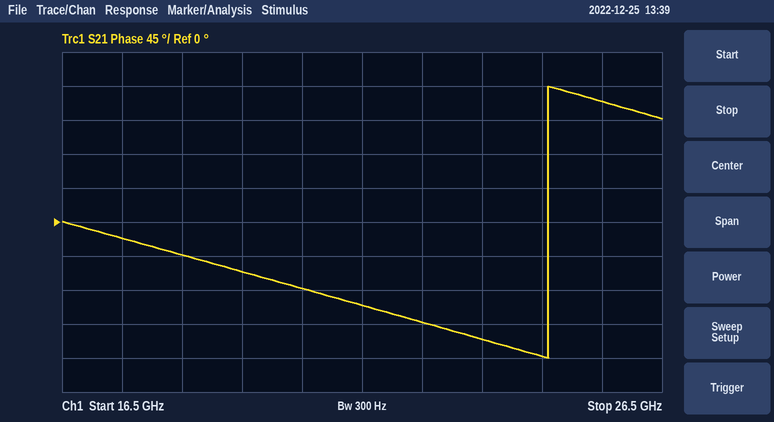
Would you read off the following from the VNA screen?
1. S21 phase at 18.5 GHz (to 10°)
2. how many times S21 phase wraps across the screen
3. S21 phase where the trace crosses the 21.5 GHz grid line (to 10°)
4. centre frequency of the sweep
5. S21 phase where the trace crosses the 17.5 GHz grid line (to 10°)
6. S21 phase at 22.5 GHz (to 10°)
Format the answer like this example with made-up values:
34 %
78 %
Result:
-40°
1
-110°
21.5 GHz
-20°
-130°
